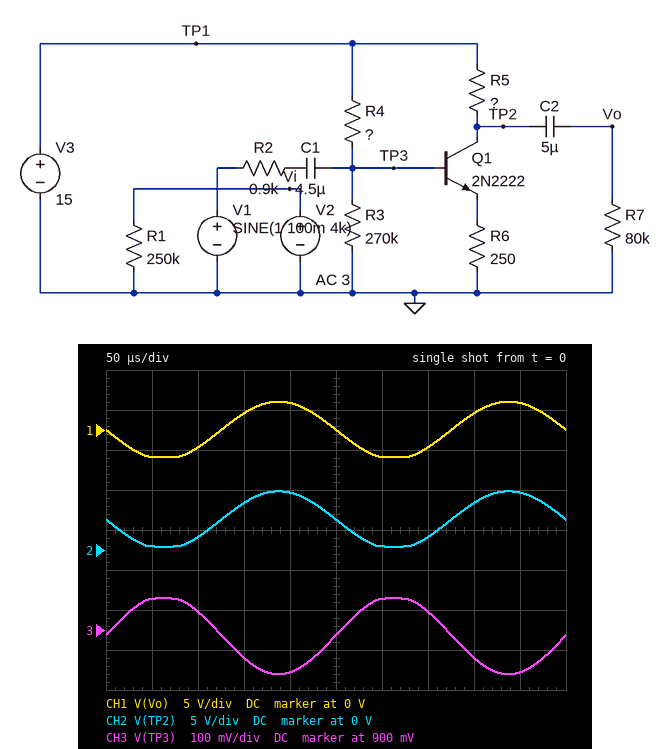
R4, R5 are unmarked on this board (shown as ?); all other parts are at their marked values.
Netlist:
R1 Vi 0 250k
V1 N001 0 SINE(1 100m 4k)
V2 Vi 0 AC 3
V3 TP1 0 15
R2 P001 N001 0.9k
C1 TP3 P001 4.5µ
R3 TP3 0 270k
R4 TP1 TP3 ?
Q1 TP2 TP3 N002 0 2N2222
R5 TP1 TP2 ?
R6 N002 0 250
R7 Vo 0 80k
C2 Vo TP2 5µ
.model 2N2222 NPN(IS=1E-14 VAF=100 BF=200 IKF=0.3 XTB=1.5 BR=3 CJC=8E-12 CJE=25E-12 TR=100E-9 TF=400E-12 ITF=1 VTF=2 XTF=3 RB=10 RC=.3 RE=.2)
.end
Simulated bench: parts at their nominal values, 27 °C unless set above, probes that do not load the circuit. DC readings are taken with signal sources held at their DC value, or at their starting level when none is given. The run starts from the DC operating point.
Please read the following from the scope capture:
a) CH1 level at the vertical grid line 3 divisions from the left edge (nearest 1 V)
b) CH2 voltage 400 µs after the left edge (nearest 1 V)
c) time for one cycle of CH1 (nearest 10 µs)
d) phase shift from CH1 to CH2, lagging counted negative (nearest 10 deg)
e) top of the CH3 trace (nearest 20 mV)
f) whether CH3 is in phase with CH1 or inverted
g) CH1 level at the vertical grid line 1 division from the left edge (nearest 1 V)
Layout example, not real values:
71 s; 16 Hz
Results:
2 V; 6 V; 250 µs; 0 deg; 980 mV; inverted; -3 V
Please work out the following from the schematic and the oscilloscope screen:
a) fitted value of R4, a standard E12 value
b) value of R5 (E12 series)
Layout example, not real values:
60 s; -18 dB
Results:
1.8 MΩ; 12 kΩ
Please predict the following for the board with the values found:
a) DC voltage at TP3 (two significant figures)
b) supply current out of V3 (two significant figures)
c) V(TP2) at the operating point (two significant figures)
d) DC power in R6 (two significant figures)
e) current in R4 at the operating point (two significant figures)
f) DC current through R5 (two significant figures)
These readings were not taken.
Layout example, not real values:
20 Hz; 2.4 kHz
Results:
890 mV; 940 µA; 3.8 V; 220 µW; 7.8 µA; 930 µA
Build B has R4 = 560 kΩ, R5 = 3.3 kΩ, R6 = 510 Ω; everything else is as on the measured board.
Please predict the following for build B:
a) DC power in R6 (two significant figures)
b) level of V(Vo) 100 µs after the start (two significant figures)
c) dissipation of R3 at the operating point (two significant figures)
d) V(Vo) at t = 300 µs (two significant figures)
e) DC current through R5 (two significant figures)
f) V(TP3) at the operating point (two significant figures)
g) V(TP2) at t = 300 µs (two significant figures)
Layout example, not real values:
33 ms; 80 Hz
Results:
4.6 mW; -350 mV; 18 µW; -570 mV; 3.0 mA; 2.2 V; 4.6 V
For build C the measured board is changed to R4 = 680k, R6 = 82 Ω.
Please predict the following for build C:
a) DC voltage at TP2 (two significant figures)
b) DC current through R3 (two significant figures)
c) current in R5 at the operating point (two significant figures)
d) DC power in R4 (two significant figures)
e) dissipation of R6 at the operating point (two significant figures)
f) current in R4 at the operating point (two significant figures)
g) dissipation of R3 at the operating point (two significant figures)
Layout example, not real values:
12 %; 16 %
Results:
200 mV; 2.8 µA; 1.2 mA; 300 µW; 130 µW; 21 µA; 2.2 µW
